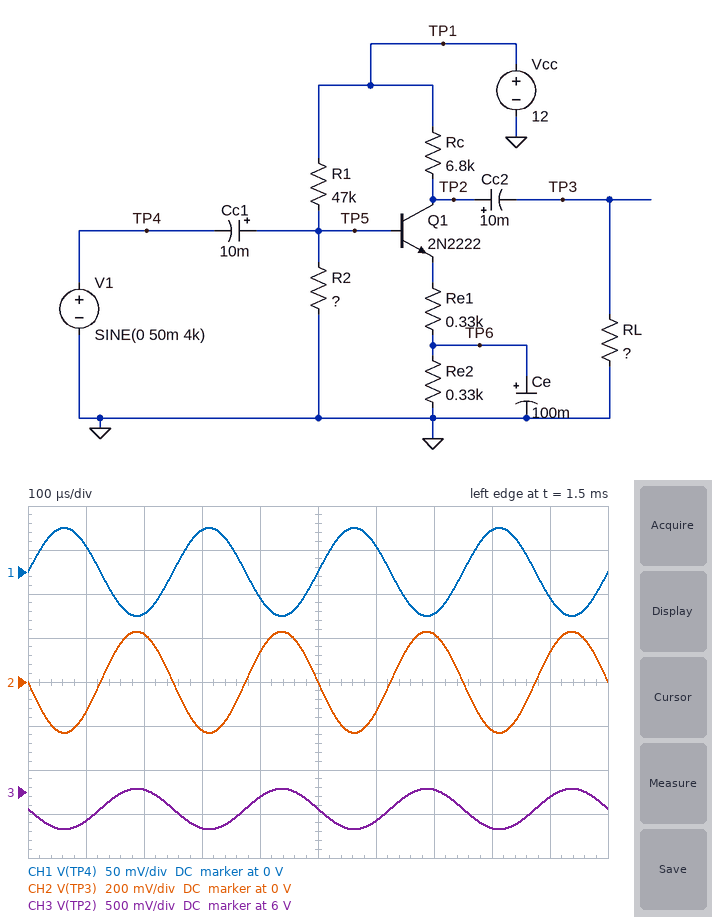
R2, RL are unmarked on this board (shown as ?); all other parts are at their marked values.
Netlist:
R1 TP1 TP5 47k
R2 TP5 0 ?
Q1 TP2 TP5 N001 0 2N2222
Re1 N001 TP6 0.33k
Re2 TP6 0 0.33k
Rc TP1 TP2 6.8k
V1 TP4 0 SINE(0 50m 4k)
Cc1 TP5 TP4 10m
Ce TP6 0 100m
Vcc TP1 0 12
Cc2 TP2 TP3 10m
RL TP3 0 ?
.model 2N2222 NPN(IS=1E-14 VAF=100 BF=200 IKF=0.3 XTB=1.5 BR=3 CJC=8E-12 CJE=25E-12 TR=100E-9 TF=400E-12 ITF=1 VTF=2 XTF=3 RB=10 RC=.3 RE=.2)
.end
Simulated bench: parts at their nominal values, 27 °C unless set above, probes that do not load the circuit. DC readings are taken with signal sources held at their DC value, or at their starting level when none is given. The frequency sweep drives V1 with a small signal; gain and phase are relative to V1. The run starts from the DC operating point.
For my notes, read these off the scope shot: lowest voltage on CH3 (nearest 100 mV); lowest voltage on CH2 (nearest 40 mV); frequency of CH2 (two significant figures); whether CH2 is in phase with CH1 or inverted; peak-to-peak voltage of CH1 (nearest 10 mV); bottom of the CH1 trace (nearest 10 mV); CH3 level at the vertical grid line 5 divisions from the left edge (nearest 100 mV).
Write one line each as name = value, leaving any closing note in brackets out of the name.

lowest voltage on CH3 = 5.6 V
lowest voltage on CH2 = -240 mV
frequency of CH2 = 4.0 kHz
whether CH2 is in phase with CH1 or inverted = inverted
peak-to-peak voltage of CH1 = 100 mV
bottom of the CH1 trace = -50 mV
CH3 level at the vertical grid line 5 divisions from the left edge = 5.8 V
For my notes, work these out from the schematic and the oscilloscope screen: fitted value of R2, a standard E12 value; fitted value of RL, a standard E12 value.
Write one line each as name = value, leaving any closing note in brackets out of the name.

fitted value of R2, a standard E12 value = 5.6 kΩ
fitted value of RL, a standard E12 value = 2.2 kΩ
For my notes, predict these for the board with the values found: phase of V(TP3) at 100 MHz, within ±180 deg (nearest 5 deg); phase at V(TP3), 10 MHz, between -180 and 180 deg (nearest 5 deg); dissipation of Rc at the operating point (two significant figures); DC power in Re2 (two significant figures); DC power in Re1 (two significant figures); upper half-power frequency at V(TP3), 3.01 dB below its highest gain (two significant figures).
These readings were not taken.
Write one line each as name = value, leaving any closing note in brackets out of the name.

phase of V(TP3) at 100 MHz, within ±180 deg = 35 deg
phase at V(TP3), 10 MHz, between -180 and 180 deg = 145 deg
dissipation of Rc at the operating point = 5.6 mW
DC power in Re2 = 280 µW
DC power in Re1 = 280 µW
upper half-power frequency at V(TP3), 3.01 dB below its highest gain = 24 MHz
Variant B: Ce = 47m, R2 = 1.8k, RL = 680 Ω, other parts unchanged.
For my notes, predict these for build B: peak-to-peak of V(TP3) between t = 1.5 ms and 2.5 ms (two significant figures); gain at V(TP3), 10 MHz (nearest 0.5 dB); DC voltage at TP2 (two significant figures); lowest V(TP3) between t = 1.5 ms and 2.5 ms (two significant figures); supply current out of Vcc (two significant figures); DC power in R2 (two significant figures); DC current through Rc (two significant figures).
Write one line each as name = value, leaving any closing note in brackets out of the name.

peak-to-peak of V(TP3) between t = 1.5 ms and 2.5 ms = 1.2 mV
gain at V(TP3), 10 MHz = -18.0 dB
DC voltage at TP2 = 12 V
lowest V(TP3) between t = 1.5 ms and 2.5 ms = -1.1 mV
supply current out of Vcc = 250 µA
DC power in R2 = 110 µW
DC current through Rc = 300 nA
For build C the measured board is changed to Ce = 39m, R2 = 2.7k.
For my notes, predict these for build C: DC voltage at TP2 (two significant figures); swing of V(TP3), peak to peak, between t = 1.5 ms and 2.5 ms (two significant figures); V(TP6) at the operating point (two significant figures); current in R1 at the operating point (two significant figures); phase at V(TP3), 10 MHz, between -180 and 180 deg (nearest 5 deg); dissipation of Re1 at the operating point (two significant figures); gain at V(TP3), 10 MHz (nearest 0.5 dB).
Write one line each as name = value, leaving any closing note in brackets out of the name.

DC voltage at TP2 = 11 V
swing of V(TP3), peak to peak, between t = 1.5 ms and 2.5 ms = 260 mV
V(TP6) at the operating point = 30 mV
current in R1 at the operating point = 240 µA
phase at V(TP3), 10 MHz, between -180 and 180 deg = 135 deg
dissipation of Re1 at the operating point = 2.8 µW
gain at V(TP3), 10 MHz = 8.0 dB
